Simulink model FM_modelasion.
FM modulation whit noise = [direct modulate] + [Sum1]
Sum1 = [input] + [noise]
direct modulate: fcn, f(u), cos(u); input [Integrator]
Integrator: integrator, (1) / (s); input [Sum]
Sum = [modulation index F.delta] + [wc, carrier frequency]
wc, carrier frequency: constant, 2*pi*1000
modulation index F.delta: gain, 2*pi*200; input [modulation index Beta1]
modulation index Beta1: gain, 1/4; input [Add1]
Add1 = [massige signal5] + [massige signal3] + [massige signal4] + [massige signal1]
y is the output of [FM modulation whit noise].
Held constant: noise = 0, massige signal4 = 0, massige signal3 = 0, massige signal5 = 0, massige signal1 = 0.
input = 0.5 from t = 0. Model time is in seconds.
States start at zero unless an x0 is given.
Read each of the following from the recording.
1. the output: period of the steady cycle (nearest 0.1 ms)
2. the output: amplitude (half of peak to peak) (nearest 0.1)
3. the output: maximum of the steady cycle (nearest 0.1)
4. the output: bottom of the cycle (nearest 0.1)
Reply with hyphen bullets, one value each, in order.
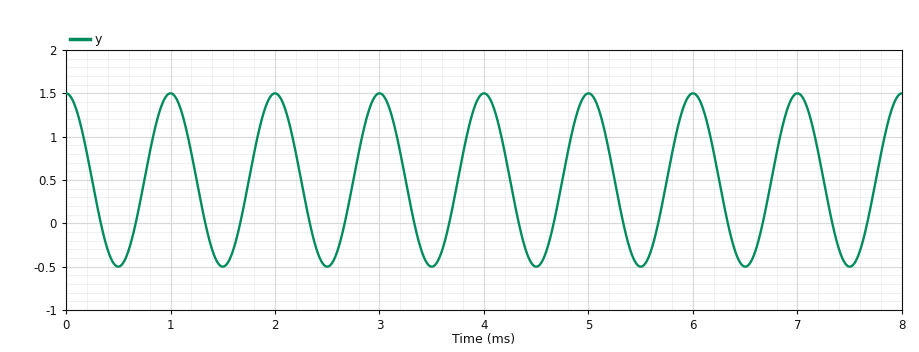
- 1.0 ms
- 1.0
- 1.5
- -0.5
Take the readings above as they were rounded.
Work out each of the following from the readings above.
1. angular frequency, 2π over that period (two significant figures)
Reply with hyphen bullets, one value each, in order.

- 6.3 rad/ms
